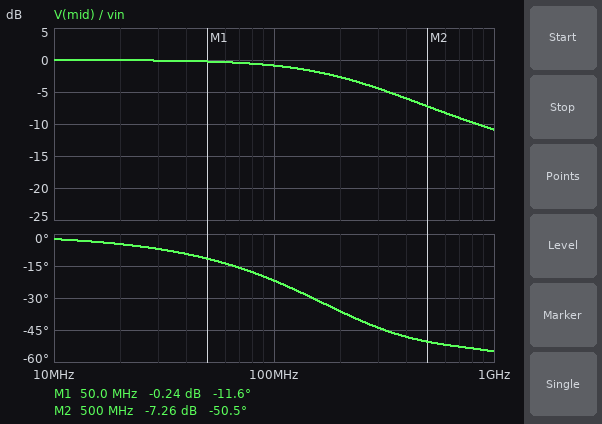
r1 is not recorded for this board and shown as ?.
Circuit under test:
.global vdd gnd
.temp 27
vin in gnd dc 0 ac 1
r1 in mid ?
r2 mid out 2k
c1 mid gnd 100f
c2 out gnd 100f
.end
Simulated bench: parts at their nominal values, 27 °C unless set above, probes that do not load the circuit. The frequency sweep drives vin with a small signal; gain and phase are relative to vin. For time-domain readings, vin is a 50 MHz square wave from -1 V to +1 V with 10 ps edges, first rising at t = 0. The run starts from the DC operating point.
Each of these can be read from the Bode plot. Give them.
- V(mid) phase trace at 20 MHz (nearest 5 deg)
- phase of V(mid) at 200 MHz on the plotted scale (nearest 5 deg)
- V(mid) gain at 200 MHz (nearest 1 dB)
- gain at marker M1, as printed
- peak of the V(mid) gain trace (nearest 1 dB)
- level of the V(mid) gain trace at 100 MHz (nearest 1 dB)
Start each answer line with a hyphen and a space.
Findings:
- -5 deg
- -35 deg
- -3 dB
- -0.24 dB
- 0 dB
- -1 dB
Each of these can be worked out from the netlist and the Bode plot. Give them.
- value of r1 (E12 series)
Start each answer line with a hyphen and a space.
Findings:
- 3.3 kΩ
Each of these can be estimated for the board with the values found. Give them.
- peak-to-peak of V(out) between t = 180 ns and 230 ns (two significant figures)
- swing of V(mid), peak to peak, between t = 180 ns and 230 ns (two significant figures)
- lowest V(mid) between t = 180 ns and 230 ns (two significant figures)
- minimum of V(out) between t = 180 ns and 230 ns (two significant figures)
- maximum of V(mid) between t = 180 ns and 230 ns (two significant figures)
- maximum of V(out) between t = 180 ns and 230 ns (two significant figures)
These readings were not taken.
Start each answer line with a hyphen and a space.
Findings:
- 2.0 V
- 2.0 V
- -1.0 V
- -1.0 V
- 1.0 V
- 1.0 V
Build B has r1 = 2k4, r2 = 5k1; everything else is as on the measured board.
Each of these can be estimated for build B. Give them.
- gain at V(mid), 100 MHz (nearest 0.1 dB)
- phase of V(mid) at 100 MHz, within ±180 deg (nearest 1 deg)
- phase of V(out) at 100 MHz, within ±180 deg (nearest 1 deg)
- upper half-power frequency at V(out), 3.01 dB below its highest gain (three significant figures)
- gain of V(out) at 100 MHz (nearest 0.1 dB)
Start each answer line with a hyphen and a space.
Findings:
- -0.7 dB
- -15 deg
- -33 deg
- 183 MHz
- -1.1 dB
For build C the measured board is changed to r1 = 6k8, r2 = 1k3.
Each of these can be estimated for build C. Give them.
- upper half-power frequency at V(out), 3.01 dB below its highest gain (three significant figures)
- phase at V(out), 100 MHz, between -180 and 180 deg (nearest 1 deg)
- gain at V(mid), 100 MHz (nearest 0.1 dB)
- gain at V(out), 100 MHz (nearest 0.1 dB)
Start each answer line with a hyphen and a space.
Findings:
- 111 MHz
- -44 deg
- -2.5 dB
- -2.6 dB
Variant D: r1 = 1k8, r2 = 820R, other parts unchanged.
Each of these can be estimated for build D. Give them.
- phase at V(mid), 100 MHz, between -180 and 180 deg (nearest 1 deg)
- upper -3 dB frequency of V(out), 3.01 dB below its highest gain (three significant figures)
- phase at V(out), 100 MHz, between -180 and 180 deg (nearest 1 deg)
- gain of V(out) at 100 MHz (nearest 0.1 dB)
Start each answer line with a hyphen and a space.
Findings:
- -13 deg
- 389 MHz
- -16 deg
- -0.3 dB
